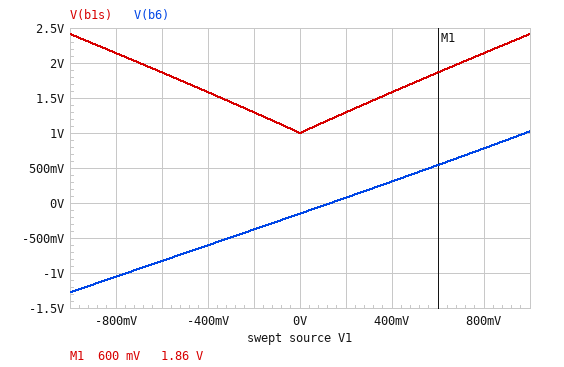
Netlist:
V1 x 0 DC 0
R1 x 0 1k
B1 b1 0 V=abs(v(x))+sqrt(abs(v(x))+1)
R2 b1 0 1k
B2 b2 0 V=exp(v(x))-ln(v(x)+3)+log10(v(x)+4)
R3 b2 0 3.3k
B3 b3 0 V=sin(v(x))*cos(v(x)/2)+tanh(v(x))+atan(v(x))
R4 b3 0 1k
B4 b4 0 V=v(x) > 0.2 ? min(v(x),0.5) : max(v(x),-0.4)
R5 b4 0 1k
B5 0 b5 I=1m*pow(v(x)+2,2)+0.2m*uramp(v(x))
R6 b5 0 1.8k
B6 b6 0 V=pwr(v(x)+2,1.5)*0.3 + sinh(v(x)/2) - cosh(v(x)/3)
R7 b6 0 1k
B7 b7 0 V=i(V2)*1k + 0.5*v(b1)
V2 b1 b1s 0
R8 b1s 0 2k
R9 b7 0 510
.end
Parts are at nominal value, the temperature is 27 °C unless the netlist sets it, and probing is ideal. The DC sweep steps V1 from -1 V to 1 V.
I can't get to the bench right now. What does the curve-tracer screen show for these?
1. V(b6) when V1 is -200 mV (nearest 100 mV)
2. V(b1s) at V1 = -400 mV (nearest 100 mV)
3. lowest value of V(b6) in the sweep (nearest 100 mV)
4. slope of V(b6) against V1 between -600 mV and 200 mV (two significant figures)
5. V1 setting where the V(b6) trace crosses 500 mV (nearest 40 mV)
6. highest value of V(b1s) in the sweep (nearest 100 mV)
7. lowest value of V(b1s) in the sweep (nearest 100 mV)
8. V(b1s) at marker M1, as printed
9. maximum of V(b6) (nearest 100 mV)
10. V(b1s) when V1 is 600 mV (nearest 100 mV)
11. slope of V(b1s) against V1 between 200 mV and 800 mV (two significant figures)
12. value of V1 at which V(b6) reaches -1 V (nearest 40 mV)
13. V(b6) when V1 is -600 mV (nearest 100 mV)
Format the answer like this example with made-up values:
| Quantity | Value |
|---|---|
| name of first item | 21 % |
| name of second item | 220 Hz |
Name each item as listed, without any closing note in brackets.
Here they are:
| Quantity | Value |
|---|---|
| V(b6) when V1 is -200 mV | -400 mV |
| V(b1s) at V1 = -400 mV | 1.6 V |
| lowest value of V(b6) in the sweep | -1.3 V |
| slope of V(b6) against V1 between -600 mV and 200 mV | 1.1 V/V |
| V1 setting where the V(b6) trace crosses 500 mV | 560 mV |
| highest value of V(b1s) in the sweep | 2.4 V |
| lowest value of V(b1s) in the sweep | 1.0 V |
| V(b1s) at marker M1, as printed | 1.86 V |
| maximum of V(b6) | 1.0 V |
| V(b1s) when V1 is 600 mV | 1.9 V |
| slope of V(b1s) against V1 between 200 mV and 800 mV | 1.4 V/V |
| value of V1 at which V(b6) reaches -1 V | -760 mV |
| V(b6) when V1 is -600 mV | -800 mV |
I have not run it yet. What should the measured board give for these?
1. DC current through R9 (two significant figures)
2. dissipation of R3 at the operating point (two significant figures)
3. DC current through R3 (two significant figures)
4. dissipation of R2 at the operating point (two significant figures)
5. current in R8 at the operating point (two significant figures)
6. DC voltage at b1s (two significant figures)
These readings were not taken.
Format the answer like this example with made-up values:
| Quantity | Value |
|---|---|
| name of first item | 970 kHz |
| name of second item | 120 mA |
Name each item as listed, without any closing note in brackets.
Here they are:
| Quantity | Value |
|---|---|
| DC current through R9 | 2.0 mA |
| dissipation of R3 at the operating point | 77 µW |
| DC current through R3 | 150 µA |
| dissipation of R2 at the operating point | 1.0 mW |
| current in R8 at the operating point | 500 µA |
| DC voltage at b1s | 1.0 V |
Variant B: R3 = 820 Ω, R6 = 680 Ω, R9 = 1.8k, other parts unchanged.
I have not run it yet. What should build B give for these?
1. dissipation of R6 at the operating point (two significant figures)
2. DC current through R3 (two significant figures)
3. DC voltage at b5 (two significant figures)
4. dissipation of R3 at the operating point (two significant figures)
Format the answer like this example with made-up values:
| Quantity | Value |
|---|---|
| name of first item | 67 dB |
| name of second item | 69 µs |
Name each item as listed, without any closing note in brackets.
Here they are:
| Quantity | Value |
|---|---|
| dissipation of R6 at the operating point | 11 mW |
| DC current through R3 | 610 µA |
| DC voltage at b5 | 2.7 V |
| dissipation of R3 at the operating point | 310 µW |
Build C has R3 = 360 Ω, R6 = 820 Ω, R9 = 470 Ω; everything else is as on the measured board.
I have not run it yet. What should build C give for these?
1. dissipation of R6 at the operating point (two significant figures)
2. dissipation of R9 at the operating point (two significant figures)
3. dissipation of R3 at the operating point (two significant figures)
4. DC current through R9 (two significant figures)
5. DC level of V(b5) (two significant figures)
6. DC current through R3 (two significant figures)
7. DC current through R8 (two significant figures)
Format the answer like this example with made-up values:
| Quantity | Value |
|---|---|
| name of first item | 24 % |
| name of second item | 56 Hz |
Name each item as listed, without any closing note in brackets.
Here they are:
| Quantity | Value |
|---|---|
| dissipation of R6 at the operating point | 13 mW |
| dissipation of R9 at the operating point | 2.1 mW |
| dissipation of R3 at the operating point | 700 µW |
| DC current through R9 | 2.1 mA |
| DC level of V(b5) | 3.3 V |
| DC current through R3 | 1.4 mA |
| DC current through R8 | 500 µA |
